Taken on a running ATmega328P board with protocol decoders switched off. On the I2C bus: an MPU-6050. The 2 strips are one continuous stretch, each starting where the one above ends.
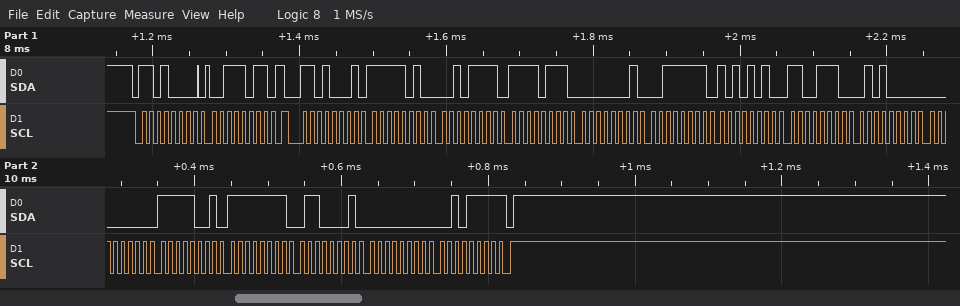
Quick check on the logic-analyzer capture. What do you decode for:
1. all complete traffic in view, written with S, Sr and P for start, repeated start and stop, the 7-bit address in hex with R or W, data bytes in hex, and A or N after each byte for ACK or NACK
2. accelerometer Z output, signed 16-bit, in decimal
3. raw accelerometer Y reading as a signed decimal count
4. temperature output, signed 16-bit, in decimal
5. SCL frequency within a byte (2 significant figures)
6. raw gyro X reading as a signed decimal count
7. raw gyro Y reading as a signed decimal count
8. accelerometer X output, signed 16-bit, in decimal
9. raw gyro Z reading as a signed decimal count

S 68W A 3B A Sr 68R A FA A 2F A F7 A 01 A 3F A AA A CE A 50 A 00 A F9 A FF A 61 A 00 A 2F N P
16298
-2303
-12720
100 kHz
249
-159
-1489
47
